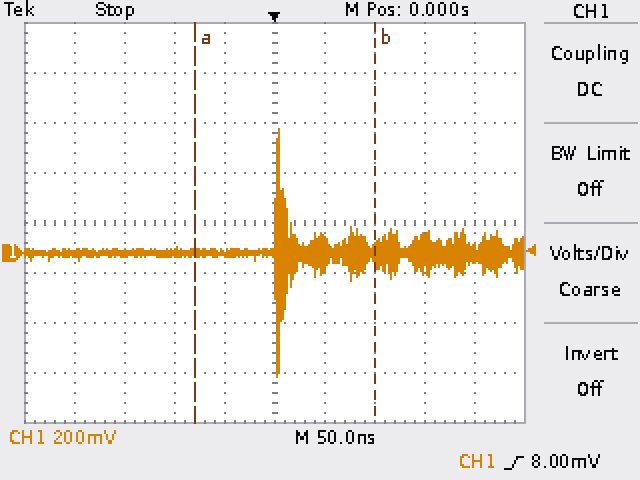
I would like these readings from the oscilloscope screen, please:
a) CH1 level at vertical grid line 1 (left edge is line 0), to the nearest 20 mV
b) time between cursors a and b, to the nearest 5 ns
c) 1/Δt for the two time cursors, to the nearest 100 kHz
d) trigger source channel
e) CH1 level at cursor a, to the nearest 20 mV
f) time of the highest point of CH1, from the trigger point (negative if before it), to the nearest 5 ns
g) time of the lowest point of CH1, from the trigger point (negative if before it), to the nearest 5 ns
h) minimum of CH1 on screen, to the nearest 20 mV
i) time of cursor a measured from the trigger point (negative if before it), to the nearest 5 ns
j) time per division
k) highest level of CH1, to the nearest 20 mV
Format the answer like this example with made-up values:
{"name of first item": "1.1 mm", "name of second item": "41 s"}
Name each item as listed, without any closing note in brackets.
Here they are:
{"CH1 level at vertical grid line 1 (left edge is line 0), to the nearest 20 mV": "0 mV", "time between cursors a and b, to the nearest 5 ns": "180 ns", "1/Δt for the two time cursors, to the nearest 100 kHz": "5.6 MHz", "trigger source channel": "CH1", "CH1 level at cursor a, to the nearest 20 mV": "0 mV", "time of the highest point of CH1, from the trigger point (negative if before it), to the nearest 5 ns": "+5 ns", "time of the lowest point of CH1, from the trigger point (negative if before it), to the nearest 5 ns": "+5 ns", "minimum of CH1 on screen, to the nearest 20 mV": "-500 mV", "time of cursor a measured from the trigger point (negative if before it), to the nearest 5 ns": "-80 ns", "time per division": "50 ns", "highest level of CH1, to the nearest 20 mV": "500 mV"}
